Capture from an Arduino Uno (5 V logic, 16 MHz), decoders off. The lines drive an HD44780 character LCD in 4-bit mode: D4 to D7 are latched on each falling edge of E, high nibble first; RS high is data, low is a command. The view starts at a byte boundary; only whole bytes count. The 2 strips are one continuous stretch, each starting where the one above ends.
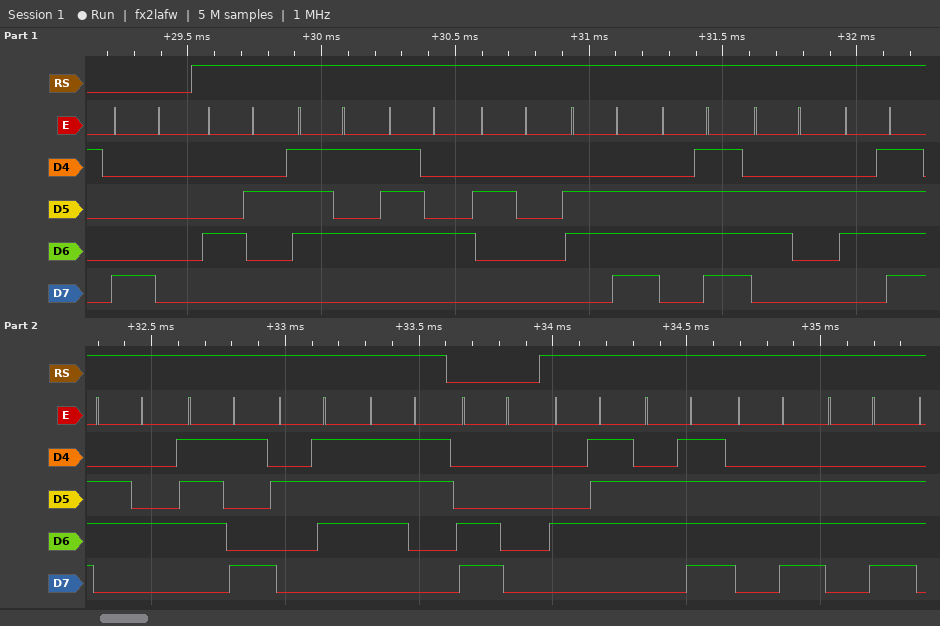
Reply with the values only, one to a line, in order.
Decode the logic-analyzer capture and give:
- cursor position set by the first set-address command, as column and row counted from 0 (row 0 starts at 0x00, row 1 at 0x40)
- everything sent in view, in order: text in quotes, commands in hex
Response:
column 0, row 0
0x80 "But nobody's" 0xC0 "Gonn"
